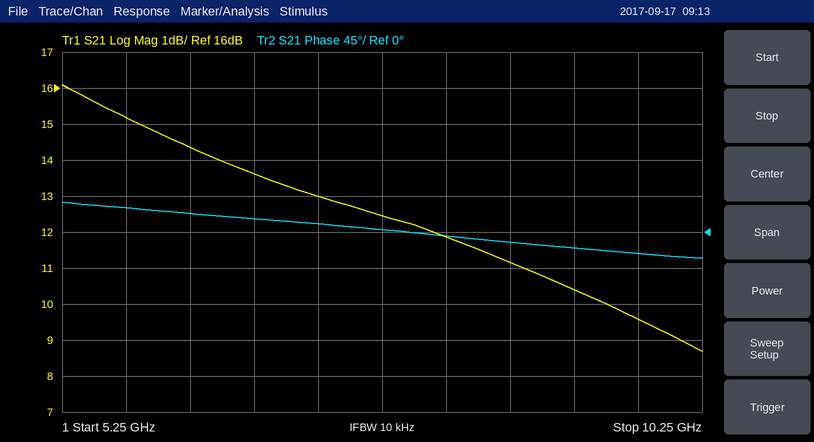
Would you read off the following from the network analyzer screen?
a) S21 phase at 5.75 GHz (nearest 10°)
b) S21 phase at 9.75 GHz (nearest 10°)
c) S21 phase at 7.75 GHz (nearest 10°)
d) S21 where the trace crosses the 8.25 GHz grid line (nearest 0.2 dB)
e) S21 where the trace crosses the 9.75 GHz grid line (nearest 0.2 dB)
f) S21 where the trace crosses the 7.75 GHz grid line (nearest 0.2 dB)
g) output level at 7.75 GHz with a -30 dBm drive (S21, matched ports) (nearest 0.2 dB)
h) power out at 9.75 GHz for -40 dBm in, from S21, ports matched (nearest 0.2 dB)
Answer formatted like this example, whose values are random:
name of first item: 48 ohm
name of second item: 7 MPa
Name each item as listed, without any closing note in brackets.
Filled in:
S21 phase at 5.75 GHz: 30°
S21 phase at 9.75 GHz: -30°
S21 phase at 7.75 GHz: 0°
S21 where the trace crosses the 8.25 GHz grid line: 11.8 dB
S21 where the trace crosses the 9.75 GHz grid line: 9.6 dB
S21 where the trace crosses the 7.75 GHz grid line: 12.4 dB
output level at 7.75 GHz with a -30 dBm drive (S21, matched ports): -17.6 dBm
power out at 9.75 GHz for -40 dBm in, from S21, ports matched: -30.4 dBm
